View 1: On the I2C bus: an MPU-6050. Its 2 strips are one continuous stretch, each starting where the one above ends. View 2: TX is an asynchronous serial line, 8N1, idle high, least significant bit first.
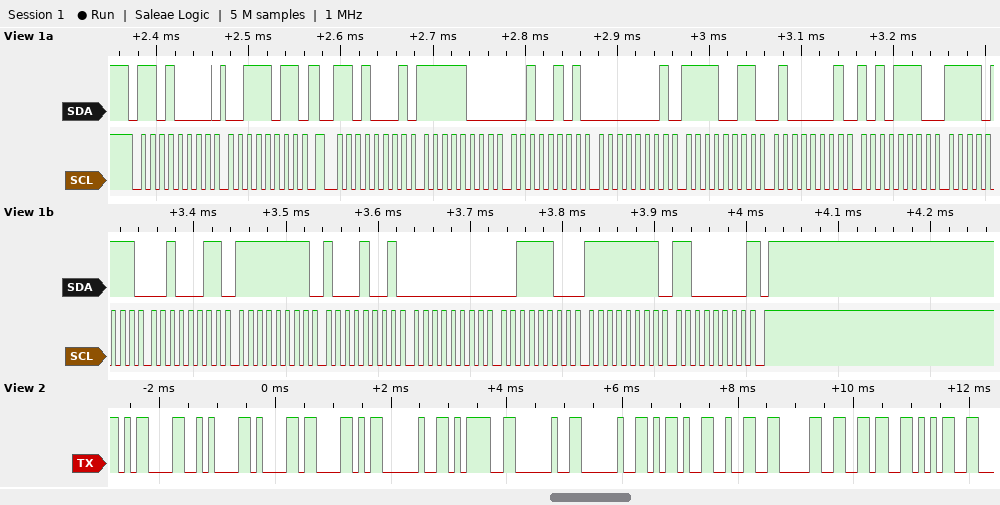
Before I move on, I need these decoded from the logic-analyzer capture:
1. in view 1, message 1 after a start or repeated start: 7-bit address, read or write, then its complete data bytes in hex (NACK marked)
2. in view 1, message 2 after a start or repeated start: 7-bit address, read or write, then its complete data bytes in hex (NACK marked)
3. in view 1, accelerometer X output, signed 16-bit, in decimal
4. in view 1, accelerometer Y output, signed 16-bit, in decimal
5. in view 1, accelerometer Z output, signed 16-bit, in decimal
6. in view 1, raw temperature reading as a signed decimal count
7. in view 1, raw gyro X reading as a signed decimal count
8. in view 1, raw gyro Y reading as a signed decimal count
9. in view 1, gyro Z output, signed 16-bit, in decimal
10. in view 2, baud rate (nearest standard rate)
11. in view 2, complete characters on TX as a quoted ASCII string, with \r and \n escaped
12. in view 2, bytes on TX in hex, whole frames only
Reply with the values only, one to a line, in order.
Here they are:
0x68 write: 3B
0x68 read: F8 25 01 F3 41 AE F7 23 FF 89 00 3C FF C0 NACK
-2011
499
16814
-2269
-119
60
-64
9600 baud
"\r\naX =  -2065"
0D 0A 61 58 20 3D 20 20 2D 32 30 36 35
